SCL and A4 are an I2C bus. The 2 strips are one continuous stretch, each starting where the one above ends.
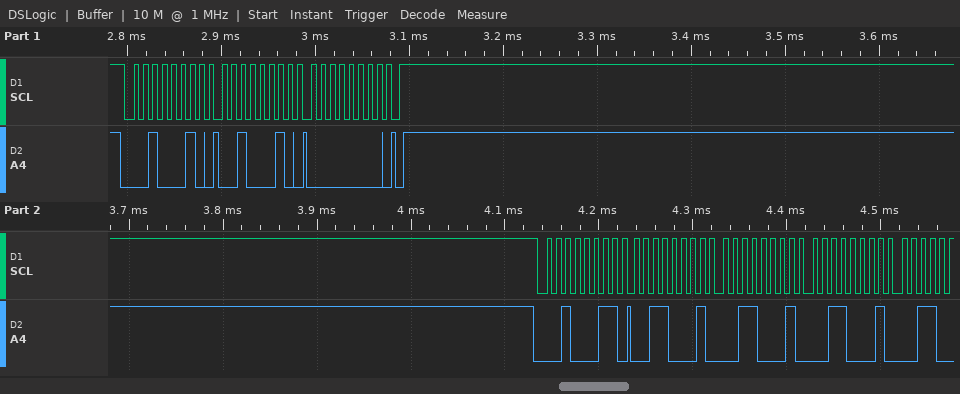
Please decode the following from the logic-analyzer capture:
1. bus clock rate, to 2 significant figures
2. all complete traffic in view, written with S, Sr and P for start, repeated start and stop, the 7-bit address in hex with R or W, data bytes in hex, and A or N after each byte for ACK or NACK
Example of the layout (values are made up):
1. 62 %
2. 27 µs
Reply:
1. 100 kHz
2. S 11W A 22 A 00 A P S 11R A 31 A 31 A 31 A
